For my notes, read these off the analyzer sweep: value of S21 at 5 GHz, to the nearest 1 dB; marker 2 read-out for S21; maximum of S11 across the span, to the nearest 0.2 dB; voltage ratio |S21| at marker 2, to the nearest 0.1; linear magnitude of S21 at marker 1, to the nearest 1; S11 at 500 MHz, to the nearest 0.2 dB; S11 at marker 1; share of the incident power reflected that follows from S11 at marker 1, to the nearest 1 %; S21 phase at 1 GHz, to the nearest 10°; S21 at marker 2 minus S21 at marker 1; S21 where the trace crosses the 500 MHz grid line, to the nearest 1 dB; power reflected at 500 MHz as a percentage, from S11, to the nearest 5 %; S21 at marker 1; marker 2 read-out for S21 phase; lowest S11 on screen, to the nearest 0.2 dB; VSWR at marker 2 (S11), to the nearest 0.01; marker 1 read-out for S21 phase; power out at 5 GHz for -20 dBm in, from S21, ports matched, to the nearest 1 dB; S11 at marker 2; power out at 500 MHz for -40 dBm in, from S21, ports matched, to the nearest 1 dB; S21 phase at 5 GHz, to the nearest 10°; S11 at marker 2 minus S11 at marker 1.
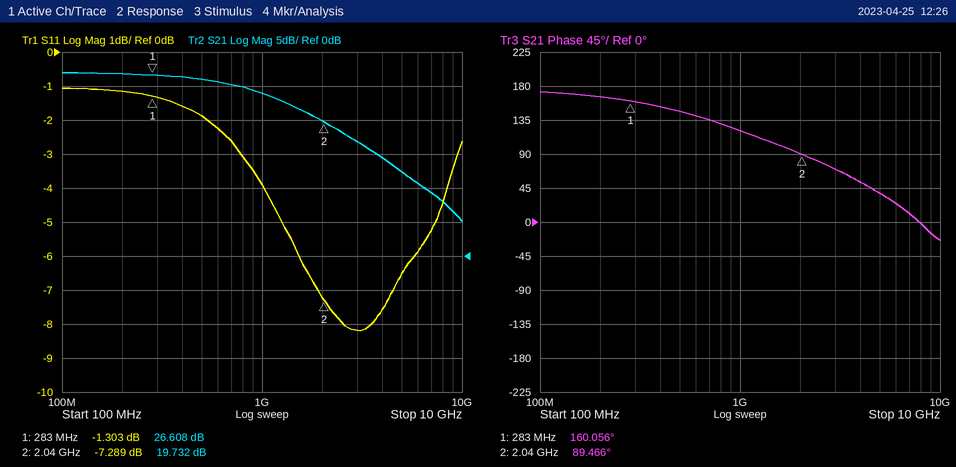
12 dB
19.732 dB
-1.0 dB
9.7
21
-1.8 dB
-1.303 dB
74 %
120°
-6.876 dB
26 dB
65 %
26.608 dB
89.466°
-8.2 dB
2.52
160.056°
-8 dBm
-7.289 dB
-14 dBm
40°
-5.986 dB
